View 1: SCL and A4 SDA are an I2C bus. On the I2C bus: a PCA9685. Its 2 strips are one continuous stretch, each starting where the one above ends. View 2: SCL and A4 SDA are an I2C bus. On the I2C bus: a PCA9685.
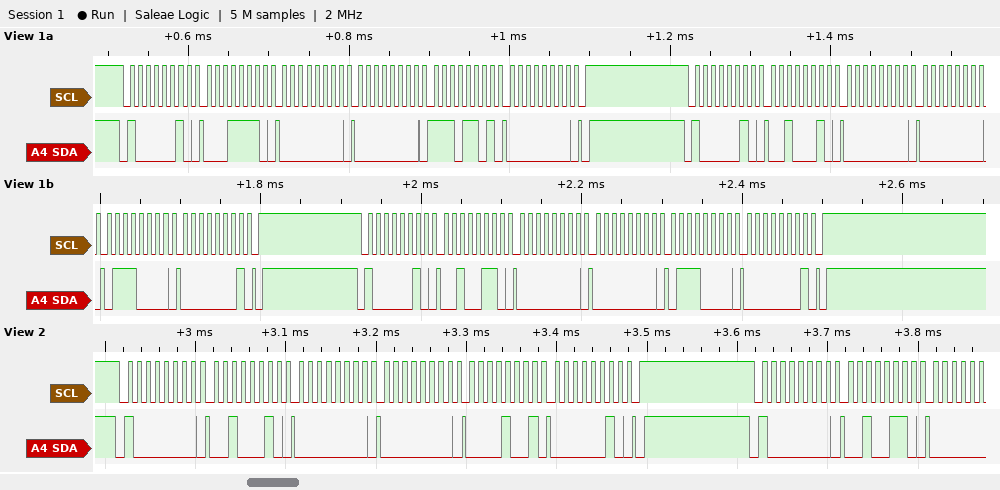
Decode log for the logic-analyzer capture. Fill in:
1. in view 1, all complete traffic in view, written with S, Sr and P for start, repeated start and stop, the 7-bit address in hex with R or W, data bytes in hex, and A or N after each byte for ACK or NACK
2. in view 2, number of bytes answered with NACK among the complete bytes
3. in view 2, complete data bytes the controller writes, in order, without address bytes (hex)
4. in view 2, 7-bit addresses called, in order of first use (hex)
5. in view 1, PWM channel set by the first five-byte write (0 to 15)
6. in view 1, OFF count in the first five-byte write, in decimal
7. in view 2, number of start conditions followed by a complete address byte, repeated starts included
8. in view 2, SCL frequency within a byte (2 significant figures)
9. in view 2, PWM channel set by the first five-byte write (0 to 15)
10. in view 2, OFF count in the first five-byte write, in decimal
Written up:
S 41W A 1E A 00 A 00 A ED A 00 A P S 41W A 22 A 00 A 00 A 70 A 01 A P S 41W A 26 A 00 A 00 A 70 A 01 A P
0
22 00 00 09 02 26
0x40
6
237
2
100 kHz
7
521
